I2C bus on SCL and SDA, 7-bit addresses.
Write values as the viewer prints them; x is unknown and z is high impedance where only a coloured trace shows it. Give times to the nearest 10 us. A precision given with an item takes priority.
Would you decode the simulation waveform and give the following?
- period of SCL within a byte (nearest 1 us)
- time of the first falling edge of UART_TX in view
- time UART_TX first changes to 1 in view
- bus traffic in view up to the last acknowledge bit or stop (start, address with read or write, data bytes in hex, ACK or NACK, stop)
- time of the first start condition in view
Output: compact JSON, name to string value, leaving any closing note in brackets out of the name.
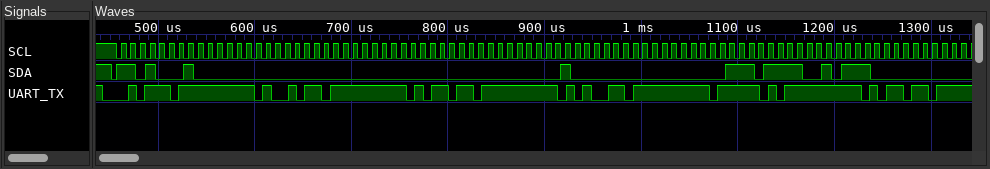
{"period of SCL within a byte": "10 us", "time of the first falling edge of UART_TX in view": "440 us", "time UART_TX first changes to 1 in view": "470 us", "bus traffic in view up to the last acknowledge bit or stop": "start, address 68 read ACK, 00 ACK, 00 ACK, 00 ACK, 00 ACK, 40 ACK, 00 ACK, EF ACK, 5C ACK", "time of the first start condition in view": "450 us"}
